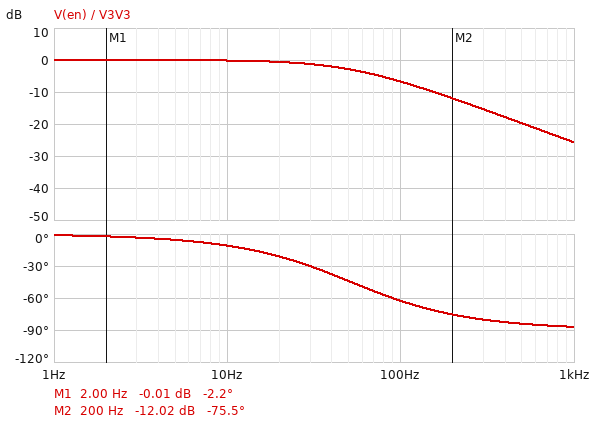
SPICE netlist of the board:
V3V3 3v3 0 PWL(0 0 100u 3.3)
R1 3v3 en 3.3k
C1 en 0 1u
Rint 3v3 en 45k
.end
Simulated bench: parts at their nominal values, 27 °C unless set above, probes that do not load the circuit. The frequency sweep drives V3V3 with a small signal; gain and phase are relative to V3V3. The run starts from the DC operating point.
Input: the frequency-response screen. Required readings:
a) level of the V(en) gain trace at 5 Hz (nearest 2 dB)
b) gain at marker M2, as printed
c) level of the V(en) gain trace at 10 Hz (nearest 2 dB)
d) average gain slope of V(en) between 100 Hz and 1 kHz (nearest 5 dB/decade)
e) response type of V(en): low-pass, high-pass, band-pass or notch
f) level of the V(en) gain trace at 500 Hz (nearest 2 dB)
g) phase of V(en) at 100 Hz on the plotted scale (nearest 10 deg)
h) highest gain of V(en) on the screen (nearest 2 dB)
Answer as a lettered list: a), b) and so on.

a) 0 dB
b) -12.02 dB
c) 0 dB
d) -20 dB/decade
e) low-pass
f) -20 dB
g) -60 deg
h) 0 dB
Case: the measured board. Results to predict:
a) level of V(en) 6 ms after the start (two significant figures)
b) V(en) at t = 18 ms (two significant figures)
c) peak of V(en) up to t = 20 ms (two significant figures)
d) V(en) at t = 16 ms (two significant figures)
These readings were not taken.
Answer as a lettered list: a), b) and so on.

a) 2.8 V
b) 3.3 V
c) 3.3 V
d) 3.3 V
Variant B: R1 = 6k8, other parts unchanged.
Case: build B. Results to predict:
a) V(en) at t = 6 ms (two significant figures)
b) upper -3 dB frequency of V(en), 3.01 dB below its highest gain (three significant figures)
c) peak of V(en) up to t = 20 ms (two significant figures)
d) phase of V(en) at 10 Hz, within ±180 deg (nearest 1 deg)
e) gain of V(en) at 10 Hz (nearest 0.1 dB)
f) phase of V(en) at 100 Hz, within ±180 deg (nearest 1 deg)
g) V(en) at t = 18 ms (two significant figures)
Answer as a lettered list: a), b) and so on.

a) 2.1 V
b) 26.9 Hz
c) 3.2 V
d) -20 deg
e) -0.6 dB
f) -75 deg
g) 3.1 V
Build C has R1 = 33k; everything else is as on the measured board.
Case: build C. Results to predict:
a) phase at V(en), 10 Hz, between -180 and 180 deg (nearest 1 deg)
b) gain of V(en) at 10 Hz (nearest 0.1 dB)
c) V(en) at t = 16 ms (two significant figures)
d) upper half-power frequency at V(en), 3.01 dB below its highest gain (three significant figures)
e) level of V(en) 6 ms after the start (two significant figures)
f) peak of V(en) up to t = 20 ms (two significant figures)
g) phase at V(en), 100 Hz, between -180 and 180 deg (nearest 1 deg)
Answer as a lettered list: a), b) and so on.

a) -50 deg
b) -3.9 dB
c) 1.9 V
d) 8.36 Hz
e) 890 mV
f) 2.1 V
g) -85 deg
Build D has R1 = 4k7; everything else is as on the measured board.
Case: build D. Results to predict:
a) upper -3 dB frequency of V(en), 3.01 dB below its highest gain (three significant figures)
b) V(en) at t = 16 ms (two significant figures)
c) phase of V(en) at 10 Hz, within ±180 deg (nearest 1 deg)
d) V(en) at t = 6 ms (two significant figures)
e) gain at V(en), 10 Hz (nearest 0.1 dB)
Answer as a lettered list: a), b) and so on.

a) 37.4 Hz
b) 3.2 V
c) -15 deg
d) 2.5 V
e) -0.3 dB
